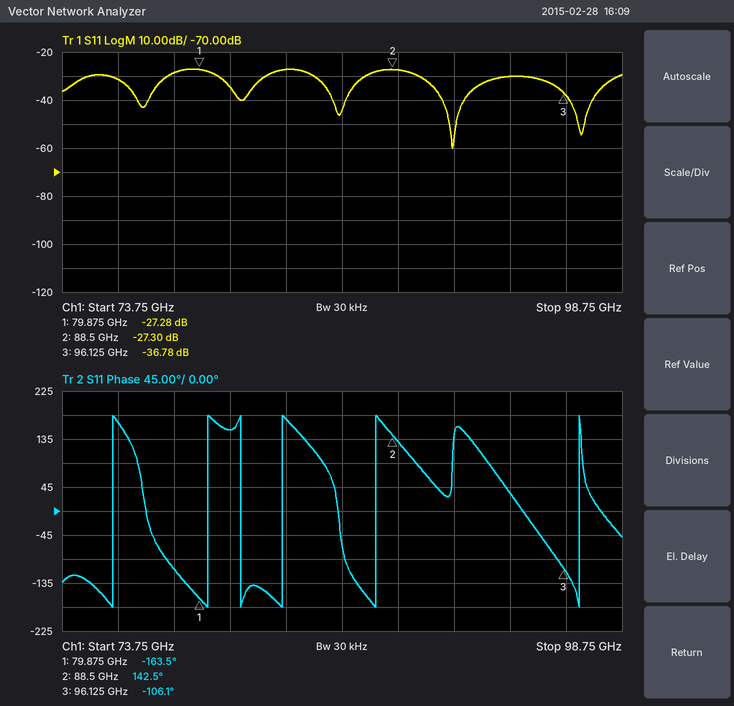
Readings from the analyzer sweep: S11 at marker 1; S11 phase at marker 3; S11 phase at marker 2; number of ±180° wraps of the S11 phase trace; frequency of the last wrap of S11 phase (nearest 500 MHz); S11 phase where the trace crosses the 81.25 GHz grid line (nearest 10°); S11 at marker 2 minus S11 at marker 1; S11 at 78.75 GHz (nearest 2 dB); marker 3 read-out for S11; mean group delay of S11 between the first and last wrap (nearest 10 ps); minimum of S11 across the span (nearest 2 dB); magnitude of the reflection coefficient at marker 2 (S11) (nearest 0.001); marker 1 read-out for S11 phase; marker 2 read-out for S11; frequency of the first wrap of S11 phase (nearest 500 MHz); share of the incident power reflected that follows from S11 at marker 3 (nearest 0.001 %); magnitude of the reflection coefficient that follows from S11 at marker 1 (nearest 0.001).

-27.28 dB
-106.1°
142.5°
6
97.0 GHz
150°
-0.02 dB
-28 dB
-36.78 dB
240 ps
-60 dB
0.043
-163.5°
-27.30 dB
76.0 GHz
0.021 %
0.043
